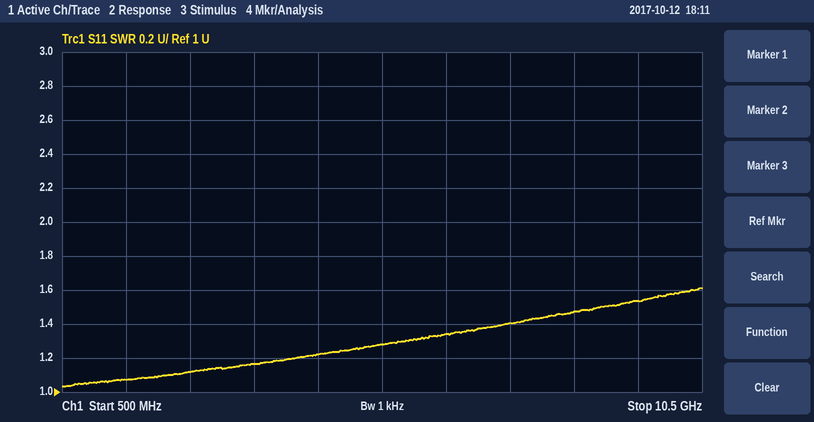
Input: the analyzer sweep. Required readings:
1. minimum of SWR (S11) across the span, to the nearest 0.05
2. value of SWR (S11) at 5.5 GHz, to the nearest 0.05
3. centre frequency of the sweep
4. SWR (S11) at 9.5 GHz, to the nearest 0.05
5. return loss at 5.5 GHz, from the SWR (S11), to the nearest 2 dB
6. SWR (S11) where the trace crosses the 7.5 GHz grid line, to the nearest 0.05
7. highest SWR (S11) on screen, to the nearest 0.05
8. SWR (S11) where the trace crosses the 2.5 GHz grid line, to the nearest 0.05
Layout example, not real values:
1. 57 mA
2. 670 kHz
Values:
1. 1.05
2. 1.30
3. 5.5 GHz
4. 1.55
5. 18 dB
6. 1.40
7. 1.60
8. 1.10
